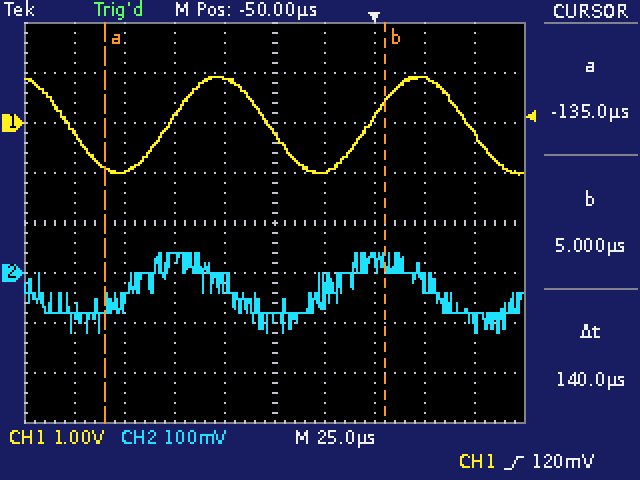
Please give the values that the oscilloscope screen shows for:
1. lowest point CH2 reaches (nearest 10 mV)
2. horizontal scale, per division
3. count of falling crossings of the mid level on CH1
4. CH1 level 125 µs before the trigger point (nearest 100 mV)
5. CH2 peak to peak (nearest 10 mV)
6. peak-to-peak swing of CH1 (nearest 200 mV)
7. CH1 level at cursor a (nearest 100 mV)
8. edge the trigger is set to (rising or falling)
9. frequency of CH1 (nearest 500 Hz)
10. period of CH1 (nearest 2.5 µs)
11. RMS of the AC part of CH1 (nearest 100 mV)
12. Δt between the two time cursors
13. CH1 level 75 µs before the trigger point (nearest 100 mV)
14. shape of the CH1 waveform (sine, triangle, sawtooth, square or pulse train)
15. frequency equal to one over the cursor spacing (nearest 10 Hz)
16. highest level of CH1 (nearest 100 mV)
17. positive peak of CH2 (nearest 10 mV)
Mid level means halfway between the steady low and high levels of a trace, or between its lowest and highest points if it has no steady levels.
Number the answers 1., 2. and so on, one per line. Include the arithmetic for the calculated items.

1. -120 mV
2. 25 µs
3. 3
4. -1.0 V
5. 40 mV − (-120 mV) = 160 mV
6. 2.0 V
7. -900 mV
8. rising
9. 1 / 100.0 µs ≈ 10.0 kHz
10. 100.0 µs
11. 2.0 V / (2√2) ≈ 707 mV, so 700 mV to the nearest 100 mV
12. 140 µs
13. 900 mV
14. sine
15. 1 / 140 µs ≈ 7.14 kHz
16. 900 mV
17. 40 mV
